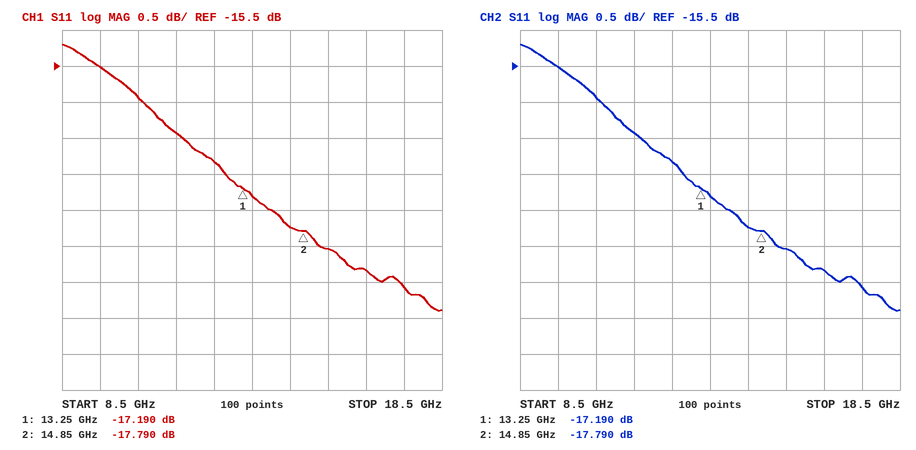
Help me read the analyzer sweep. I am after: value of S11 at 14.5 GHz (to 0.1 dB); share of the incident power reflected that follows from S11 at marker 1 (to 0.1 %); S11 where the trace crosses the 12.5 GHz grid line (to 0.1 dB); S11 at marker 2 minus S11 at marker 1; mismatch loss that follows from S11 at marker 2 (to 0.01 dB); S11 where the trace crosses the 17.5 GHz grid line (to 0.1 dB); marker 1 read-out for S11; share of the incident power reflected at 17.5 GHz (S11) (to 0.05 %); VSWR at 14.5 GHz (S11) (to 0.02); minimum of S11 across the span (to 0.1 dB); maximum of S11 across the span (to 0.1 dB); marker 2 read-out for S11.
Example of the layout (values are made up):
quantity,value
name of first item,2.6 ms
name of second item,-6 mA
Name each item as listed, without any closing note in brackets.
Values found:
quantity,value
value of S11 at 14.5 GHz,-17.7 dB
share of the incident power reflected that follows from S11 at marker 1,1.9 %
S11 where the trace crosses the 12.5 GHz grid line,-16.8 dB
S11 at marker 2 minus S11 at marker 1,-0.600 dB
mismatch loss that follows from S11 at marker 2,0.07 dB
S11 where the trace crosses the 17.5 GHz grid line,-18.6 dB
marker 1 read-out for S11,-17.190 dB
share of the incident power reflected at 17.5 GHz (S11),1.40 %
VSWR at 14.5 GHz (S11),1.30
minimum of S11 across the span,-18.9 dB
maximum of S11 across the span,-15.2 dB
marker 2 read-out for S11,-17.790 dB
